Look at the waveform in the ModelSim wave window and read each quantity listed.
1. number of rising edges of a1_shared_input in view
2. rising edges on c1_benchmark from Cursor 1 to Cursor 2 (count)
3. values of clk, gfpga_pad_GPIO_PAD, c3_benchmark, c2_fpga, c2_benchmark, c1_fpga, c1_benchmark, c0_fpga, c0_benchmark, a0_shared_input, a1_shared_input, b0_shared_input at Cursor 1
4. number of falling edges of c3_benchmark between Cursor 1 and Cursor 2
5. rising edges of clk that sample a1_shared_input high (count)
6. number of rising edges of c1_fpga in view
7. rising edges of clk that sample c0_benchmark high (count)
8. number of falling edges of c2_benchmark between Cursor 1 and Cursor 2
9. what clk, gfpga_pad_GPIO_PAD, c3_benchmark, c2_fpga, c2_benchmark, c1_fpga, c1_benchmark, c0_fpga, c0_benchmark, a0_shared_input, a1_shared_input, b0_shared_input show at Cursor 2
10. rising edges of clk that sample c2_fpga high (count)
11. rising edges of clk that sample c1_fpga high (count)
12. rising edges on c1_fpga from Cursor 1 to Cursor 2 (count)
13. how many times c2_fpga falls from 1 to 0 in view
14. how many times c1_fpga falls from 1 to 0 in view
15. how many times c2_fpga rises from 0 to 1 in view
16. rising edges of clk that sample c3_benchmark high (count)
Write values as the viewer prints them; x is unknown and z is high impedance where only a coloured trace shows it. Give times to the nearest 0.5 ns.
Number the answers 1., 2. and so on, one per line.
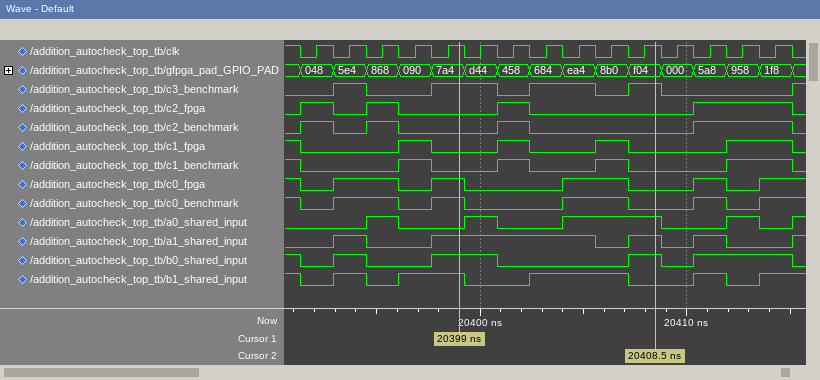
1. 5
2. 2
3. clk=1, gfpga_pad_GPIO_PAD=7a4, c3_benchmark=1, c2_fpga=0, c2_benchmark=0, c1_fpga=0, c1_benchmark=0, c0_fpga=1, c0_benchmark=1, a0_shared_input=0, a1_shared_input=1, b0_shared_input=1
4. 2
5. 8
6. 4
7. 7
8. 1
9. clk=1, gfpga_pad_GPIO_PAD=f04, c3_benchmark=1, c2_fpga=0, c2_benchmark=0, c1_fpga=0, c1_benchmark=0, c0_fpga=0, c0_benchmark=0, a0_shared_input=1, a1_shared_input=1, b0_shared_input=1
10. 6
11. 5
12. 2
13. 4
14. 5
15. 4
16. 6
